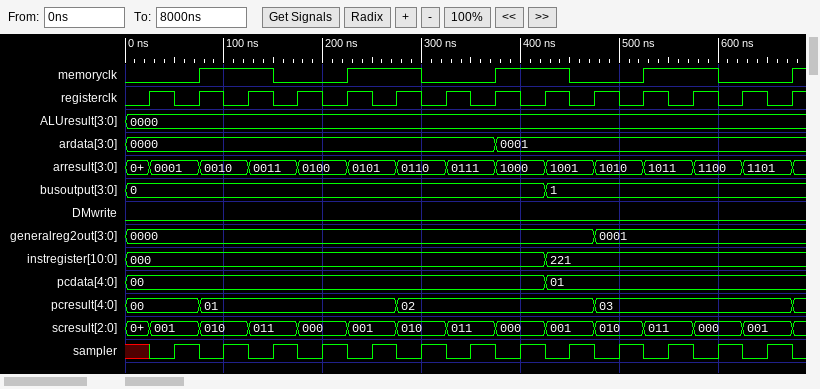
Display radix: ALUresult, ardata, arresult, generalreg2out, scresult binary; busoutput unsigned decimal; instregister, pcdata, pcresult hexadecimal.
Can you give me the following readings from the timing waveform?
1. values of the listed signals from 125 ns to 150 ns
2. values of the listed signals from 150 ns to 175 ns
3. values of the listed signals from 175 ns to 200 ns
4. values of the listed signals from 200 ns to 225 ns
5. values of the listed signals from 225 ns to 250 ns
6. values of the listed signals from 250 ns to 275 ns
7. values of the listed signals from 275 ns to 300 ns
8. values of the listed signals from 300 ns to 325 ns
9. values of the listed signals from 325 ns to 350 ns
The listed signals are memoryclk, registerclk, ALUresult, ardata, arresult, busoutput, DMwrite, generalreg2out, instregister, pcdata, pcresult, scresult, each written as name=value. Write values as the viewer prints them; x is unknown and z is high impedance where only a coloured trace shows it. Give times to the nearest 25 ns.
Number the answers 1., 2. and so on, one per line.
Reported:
1. memoryclk=1, registerclk=1, ALUresult=0000, ardata=0000, arresult=0011, busoutput=0, DMwrite=0, generalreg2out=0000, instregister=000, pcdata=00, pcresult=01, scresult=011
2. memoryclk=0, registerclk=0, ALUresult=0000, ardata=0000, arresult=0011, busoutput=0, DMwrite=0, generalreg2out=0000, instregister=000, pcdata=00, pcresult=01, scresult=011
3. memoryclk=0, registerclk=1, ALUresult=0000, ardata=0000, arresult=0100, busoutput=0, DMwrite=0, generalreg2out=0000, instregister=000, pcdata=00, pcresult=01, scresult=000
4. memoryclk=0, registerclk=0, ALUresult=0000, ardata=0000, arresult=0100, busoutput=0, DMwrite=0, generalreg2out=0000, instregister=000, pcdata=00, pcresult=01, scresult=000
5. memoryclk=1, registerclk=1, ALUresult=0000, ardata=0000, arresult=0101, busoutput=0, DMwrite=0, generalreg2out=0000, instregister=000, pcdata=00, pcresult=01, scresult=001
6. memoryclk=1, registerclk=0, ALUresult=0000, ardata=0000, arresult=0101, busoutput=0, DMwrite=0, generalreg2out=0000, instregister=000, pcdata=00, pcresult=01, scresult=001
7. memoryclk=1, registerclk=1, ALUresult=0000, ardata=0000, arresult=0110, busoutput=0, DMwrite=0, generalreg2out=0000, instregister=000, pcdata=00, pcresult=02, scresult=010
8. memoryclk=0, registerclk=0, ALUresult=0000, ardata=0000, arresult=0110, busoutput=0, DMwrite=0, generalreg2out=0000, instregister=000, pcdata=00, pcresult=02, scresult=010
9. memoryclk=0, registerclk=1, ALUresult=0000, ardata=0000, arresult=0111, busoutput=0, DMwrite=0, generalreg2out=0000, instregister=000, pcdata=00, pcresult=02, scresult=011
